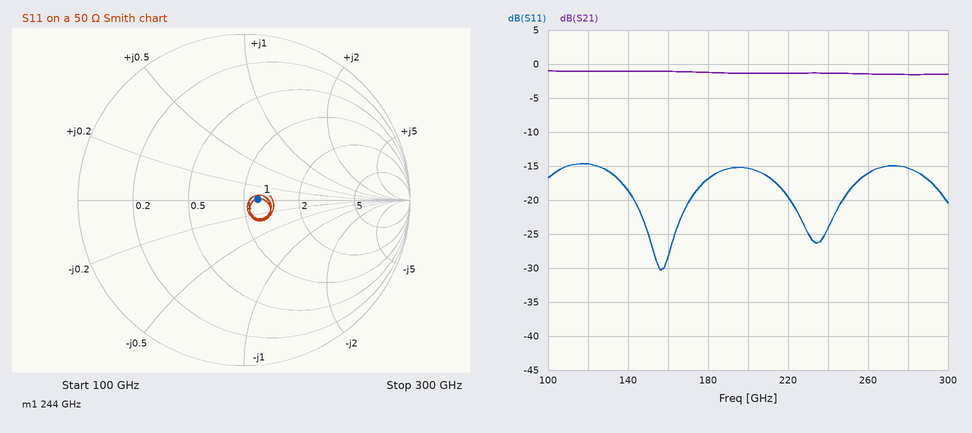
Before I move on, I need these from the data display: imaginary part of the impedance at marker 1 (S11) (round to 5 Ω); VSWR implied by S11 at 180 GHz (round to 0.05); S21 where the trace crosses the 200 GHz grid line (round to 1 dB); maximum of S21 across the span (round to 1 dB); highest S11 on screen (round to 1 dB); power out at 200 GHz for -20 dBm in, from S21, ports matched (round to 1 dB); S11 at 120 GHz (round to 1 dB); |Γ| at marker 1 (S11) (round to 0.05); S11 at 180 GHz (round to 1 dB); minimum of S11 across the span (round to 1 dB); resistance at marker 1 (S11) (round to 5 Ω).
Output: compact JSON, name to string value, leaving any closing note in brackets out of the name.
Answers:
{"imaginary part of the impedance at marker 1 (S11)": "0 Ω", "VSWR implied by S11 at 180 GHz": "1.35", "S21 where the trace crosses the 200 GHz grid line": "-1 dB", "maximum of S21 across the span": "-1 dB", "highest S11 on screen": "-15 dB", "power out at 200 GHz for -20 dBm in, from S21, ports matched": "-21 dBm", "S11 at 120 GHz": "-15 dB", "|Γ| at marker 1 (S11)": "0.10", "S11 at 180 GHz": "-17 dB", "minimum of S11 across the span": "-30 dB", "resistance at marker 1 (S11)": "60 Ω"}
